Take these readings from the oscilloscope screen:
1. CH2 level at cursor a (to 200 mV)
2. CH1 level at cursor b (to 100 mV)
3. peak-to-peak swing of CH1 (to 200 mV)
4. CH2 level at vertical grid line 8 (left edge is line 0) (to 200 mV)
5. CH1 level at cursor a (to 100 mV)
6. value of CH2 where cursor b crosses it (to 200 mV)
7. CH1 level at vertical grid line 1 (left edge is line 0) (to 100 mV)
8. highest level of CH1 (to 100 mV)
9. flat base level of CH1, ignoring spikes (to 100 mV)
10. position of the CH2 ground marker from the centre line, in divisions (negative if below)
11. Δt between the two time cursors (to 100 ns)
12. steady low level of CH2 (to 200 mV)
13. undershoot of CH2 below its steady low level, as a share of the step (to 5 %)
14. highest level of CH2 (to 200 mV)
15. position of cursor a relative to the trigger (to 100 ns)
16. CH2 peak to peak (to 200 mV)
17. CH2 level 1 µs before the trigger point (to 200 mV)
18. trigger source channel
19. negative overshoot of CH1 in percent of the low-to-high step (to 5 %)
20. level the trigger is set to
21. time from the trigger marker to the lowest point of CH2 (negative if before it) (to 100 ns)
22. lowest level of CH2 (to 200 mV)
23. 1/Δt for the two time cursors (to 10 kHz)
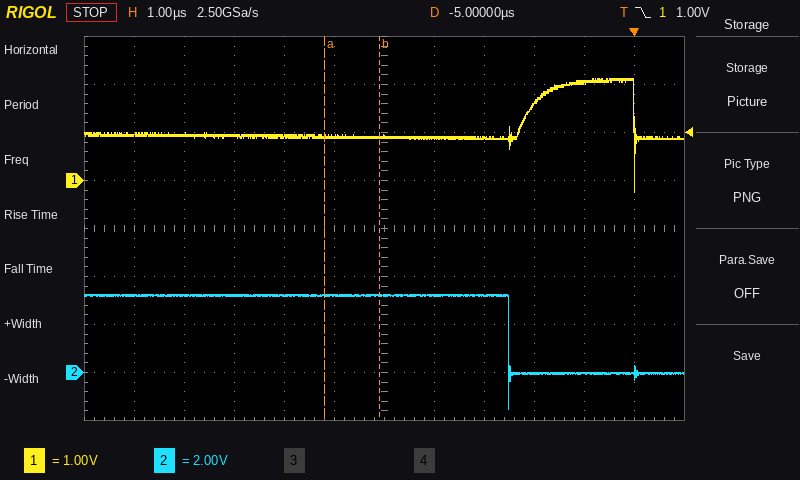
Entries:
3.2 V
900 mV
2.4 V
3.2 V
900 mV
3.2 V
1.0 V
2.1 V
900 mV
-3.0 div
1.1 µs
0.0 V
45 %
3.2 V
-6.2 µs
4.8 V
0.0 V
CH1
100 %
1.00 V
-2.5 µs
-1.6 V
910 kHz
